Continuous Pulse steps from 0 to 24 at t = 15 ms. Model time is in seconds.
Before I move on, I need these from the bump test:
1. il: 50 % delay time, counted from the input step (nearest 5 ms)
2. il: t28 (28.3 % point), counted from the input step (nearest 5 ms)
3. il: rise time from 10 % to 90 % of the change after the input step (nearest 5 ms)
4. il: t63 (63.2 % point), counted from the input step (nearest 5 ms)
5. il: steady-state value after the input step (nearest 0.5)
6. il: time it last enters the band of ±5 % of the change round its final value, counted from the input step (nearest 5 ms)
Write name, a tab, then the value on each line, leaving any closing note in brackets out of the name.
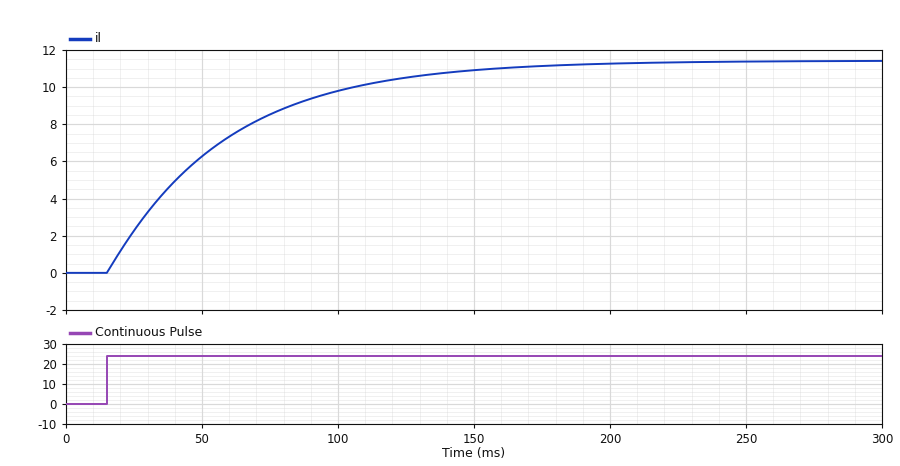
il: 50 % delay time, counted from the input step	30 ms
il: t28 (28.3 % point), counted from the input step	15 ms
il: rise time from 10 % to 90 % of the change after the input step	95 ms
il: t63 (63.2 % point), counted from the input step	45 ms
il: steady-state value after the input step	11.5
il: time it last enters the band of ±5 % of the change round its final value, counted from the input step	130 ms
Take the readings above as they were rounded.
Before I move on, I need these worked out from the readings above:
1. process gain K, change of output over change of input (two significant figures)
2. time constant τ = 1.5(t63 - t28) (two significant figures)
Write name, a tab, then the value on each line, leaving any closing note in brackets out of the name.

process gain K, change of output over change of input	0.48
time constant τ = 1.5(t63 - t28)	45 ms
